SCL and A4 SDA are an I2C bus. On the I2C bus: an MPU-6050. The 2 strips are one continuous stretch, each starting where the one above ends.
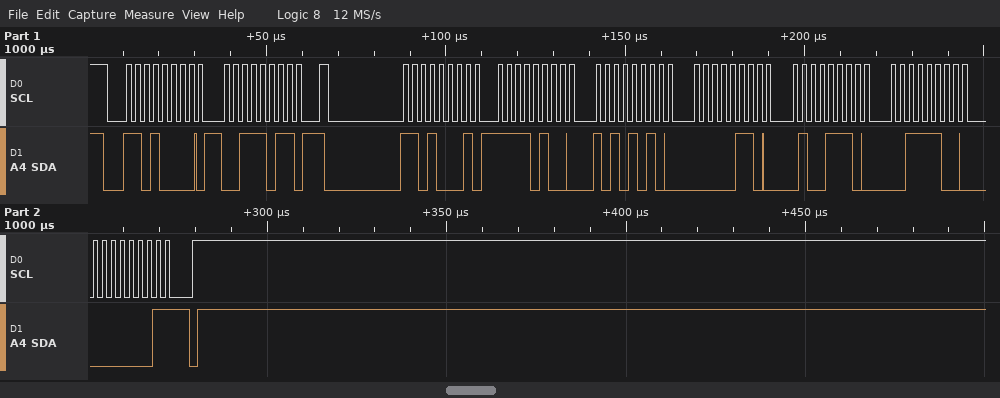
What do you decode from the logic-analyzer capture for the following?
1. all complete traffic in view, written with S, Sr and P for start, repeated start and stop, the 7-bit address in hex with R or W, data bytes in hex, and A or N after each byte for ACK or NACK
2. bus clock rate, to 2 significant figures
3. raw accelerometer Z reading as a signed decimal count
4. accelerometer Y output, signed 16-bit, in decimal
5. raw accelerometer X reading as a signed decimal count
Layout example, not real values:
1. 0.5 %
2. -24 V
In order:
1. S 68W A 3B A Sr 68R A F4 A AA A 06 A 4E A 3C A 01 N P
2. 400 kHz
3. 15361
4. 1614
5. -2902
